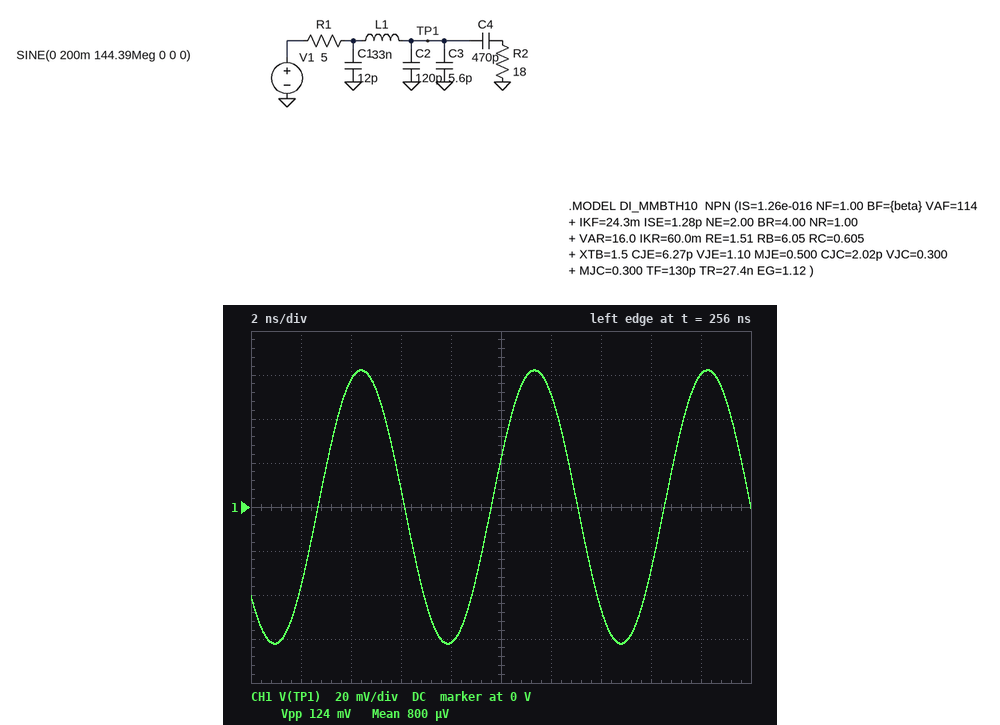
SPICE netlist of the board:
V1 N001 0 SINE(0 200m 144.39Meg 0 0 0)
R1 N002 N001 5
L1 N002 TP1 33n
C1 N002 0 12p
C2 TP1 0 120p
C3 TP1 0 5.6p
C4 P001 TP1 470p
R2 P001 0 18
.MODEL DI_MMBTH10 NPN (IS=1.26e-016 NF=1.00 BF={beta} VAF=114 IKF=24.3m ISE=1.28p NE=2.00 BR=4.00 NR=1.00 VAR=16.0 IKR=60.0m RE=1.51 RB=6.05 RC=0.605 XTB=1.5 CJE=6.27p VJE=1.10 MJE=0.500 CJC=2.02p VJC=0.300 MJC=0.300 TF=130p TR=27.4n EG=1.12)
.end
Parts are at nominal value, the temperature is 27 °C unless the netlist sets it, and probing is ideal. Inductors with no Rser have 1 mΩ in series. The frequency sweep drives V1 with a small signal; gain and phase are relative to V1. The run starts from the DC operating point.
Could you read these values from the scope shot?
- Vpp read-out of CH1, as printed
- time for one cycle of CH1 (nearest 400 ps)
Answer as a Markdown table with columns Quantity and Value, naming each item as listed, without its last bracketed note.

| Quantity | Value |
|---|---|
| Vpp read-out of CH1, as printed | 124 mV |
| time for one cycle of CH1 | 6.8 ns |
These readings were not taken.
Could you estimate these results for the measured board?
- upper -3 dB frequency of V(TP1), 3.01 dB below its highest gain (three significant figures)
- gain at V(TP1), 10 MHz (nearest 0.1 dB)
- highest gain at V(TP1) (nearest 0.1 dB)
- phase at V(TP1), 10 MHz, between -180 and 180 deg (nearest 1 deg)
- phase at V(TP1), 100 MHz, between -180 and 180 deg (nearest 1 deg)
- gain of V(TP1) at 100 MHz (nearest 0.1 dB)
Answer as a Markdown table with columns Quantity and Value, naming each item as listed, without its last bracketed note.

| Quantity | Value |
|---|---|
| upper -3 dB frequency of V(TP1), 3.01 dB below its highest gain | 89.8 MHz |
| gain at V(TP1), 10 MHz | -0.1 dB |
| highest gain at V(TP1) | 0 dB |
| phase at V(TP1), 10 MHz, between -180 and 180 deg | -10 deg |
| phase at V(TP1), 100 MHz, between -180 and 180 deg | -112 deg |
| gain of V(TP1) at 100 MHz | -4.3 dB |
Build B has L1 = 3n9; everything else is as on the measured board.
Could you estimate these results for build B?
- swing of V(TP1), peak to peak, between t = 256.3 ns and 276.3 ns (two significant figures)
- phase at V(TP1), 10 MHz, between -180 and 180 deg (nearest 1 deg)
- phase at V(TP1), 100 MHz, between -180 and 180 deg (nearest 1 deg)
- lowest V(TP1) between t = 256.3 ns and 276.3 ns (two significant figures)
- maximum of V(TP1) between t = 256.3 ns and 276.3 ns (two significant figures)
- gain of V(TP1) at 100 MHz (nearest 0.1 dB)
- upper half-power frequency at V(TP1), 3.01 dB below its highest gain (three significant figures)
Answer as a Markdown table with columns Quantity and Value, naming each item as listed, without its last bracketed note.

| Quantity | Value |
|---|---|
| swing of V(TP1), peak to peak, between t = 256.3 ns and 276.3 ns | 340 mV |
| phase at V(TP1), 10 MHz, between -180 and 180 deg | -9 deg |
| phase at V(TP1), 100 MHz, between -180 and 180 deg | -30 deg |
| lowest V(TP1) between t = 256.3 ns and 276.3 ns | -170 mV |
| maximum of V(TP1) between t = 256.3 ns and 276.3 ns | 170 mV |
| gain of V(TP1) at 100 MHz | -1.6 dB |
| upper half-power frequency at V(TP1), 3.01 dB below its highest gain | 269 MHz |
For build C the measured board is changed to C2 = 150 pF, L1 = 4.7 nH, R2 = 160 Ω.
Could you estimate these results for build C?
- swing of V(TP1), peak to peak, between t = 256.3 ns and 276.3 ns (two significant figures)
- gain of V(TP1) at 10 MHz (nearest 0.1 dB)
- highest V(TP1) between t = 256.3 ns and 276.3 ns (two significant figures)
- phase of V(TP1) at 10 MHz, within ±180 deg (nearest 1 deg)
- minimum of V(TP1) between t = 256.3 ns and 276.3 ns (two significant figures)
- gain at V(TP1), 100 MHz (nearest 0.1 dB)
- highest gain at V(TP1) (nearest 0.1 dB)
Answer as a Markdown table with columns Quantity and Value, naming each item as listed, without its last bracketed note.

| Quantity | Value |
|---|---|
| swing of V(TP1), peak to peak, between t = 256.3 ns and 276.3 ns | 460 mV |
| gain of V(TP1) at 10 MHz | -0.2 dB |
| highest V(TP1) between t = 256.3 ns and 276.3 ns | 230 mV |
| phase of V(TP1) at 10 MHz, within ±180 deg | -3 deg |
| minimum of V(TP1) between t = 256.3 ns and 276.3 ns | -230 mV |
| gain at V(TP1), 100 MHz | 0.8 dB |
| highest gain at V(TP1) | 1.2 dB |
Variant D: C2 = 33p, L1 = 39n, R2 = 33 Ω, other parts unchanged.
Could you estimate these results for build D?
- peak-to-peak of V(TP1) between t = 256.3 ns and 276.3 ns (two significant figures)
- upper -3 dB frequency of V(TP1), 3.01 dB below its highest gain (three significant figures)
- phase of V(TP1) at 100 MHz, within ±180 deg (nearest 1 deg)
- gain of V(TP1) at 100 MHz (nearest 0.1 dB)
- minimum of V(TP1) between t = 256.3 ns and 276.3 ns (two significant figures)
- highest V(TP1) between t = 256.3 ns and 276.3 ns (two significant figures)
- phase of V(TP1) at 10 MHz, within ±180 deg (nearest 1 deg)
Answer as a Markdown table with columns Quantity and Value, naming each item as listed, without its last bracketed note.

| Quantity | Value |
|---|---|
| peak-to-peak of V(TP1) between t = 256.3 ns and 276.3 ns | 320 mV |
| upper -3 dB frequency of V(TP1), 3.01 dB below its highest gain | 156 MHz |
| phase of V(TP1) at 100 MHz, within ±180 deg | -63 deg |
| gain of V(TP1) at 100 MHz | 0.1 dB |
| minimum of V(TP1) between t = 256.3 ns and 276.3 ns | -160 mV |
| highest V(TP1) between t = 256.3 ns and 276.3 ns | 160 mV |
| phase of V(TP1) at 10 MHz, within ±180 deg | -7 deg |
